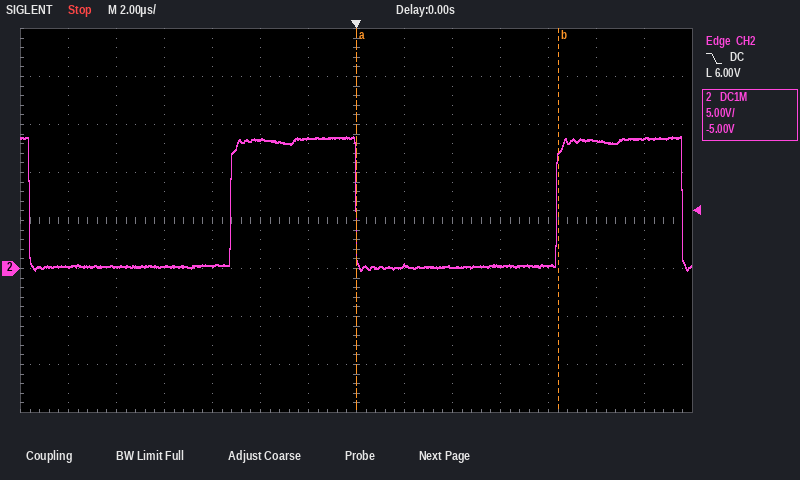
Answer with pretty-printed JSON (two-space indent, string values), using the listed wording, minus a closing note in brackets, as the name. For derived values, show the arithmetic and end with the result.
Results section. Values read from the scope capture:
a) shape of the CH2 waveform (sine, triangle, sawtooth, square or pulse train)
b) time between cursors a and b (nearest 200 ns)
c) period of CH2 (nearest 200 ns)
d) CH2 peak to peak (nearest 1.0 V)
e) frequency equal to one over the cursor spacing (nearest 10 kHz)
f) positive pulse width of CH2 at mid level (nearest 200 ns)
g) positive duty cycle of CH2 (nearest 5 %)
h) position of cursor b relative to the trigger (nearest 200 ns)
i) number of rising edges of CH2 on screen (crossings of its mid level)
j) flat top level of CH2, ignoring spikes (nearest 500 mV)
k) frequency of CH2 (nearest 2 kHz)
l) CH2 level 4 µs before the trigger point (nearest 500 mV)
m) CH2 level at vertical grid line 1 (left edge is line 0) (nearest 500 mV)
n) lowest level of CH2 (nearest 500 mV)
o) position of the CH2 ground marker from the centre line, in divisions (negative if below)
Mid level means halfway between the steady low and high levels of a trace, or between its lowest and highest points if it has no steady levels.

{
  "shape of the CH2 waveform": "pulse train",
  "time between cursors a and b": "8.4 µs",
  "period of CH2": "13.6 µs",
  "CH2 peak to peak": "14.0 V",
  "frequency equal to one over the cursor spacing": "1 / 8.4 µs ≈ 120 kHz",
  "positive pulse width of CH2 at mid level": "5.2 µs",
  "positive duty cycle of CH2": "5.2 µs / 13.6 µs ≈ 38.2 %, so 40 % to the nearest 5 %",
  "position of cursor b relative to the trigger": "+8.4 µs",
  "number of rising edges of CH2 on screen": "2",
  "flat top level of CH2, ignoring spikes": "13.5 V",
  "frequency of CH2": "1 / 13.6 µs ≈ 74 kHz",
  "CH2 level 4 µs before the trigger point": "13.5 V",
  "CH2 level at vertical grid line 1 (left edge is line 0)": "0.0 V",
  "lowest level of CH2": "0.0 V",
  "position of the CH2 ground marker from the centre line, in divisions": "-1.0 div"
}
